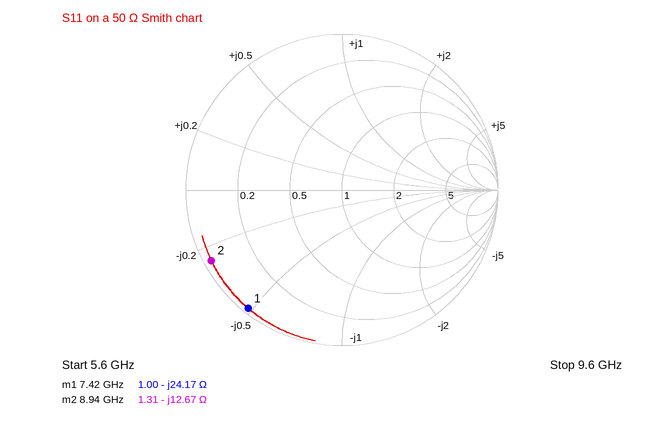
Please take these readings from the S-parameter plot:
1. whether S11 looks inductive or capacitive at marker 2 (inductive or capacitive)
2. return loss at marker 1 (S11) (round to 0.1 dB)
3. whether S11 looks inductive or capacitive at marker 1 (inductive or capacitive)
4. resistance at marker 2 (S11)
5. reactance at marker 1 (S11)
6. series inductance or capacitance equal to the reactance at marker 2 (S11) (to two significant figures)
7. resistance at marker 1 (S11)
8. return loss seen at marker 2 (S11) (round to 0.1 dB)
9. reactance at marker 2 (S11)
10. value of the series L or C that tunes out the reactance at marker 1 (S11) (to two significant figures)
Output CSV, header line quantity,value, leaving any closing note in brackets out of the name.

quantity,value
whether S11 looks inductive or capacitive at marker 2,capacitive
return loss at marker 1 (S11),0.3 dB
whether S11 looks inductive or capacitive at marker 1,capacitive
resistance at marker 2,1.31 Ω
reactance at marker 1,-24.17 Ω
series inductance or capacitance equal to the reactance at marker 2 (S11),1.4 pF
resistance at marker 1,1.00 Ω
return loss seen at marker 2 (S11),0.4 dB
reactance at marker 2,-12.67 Ω
value of the series L or C that tunes out the reactance at marker 1 (S11),520 pH
